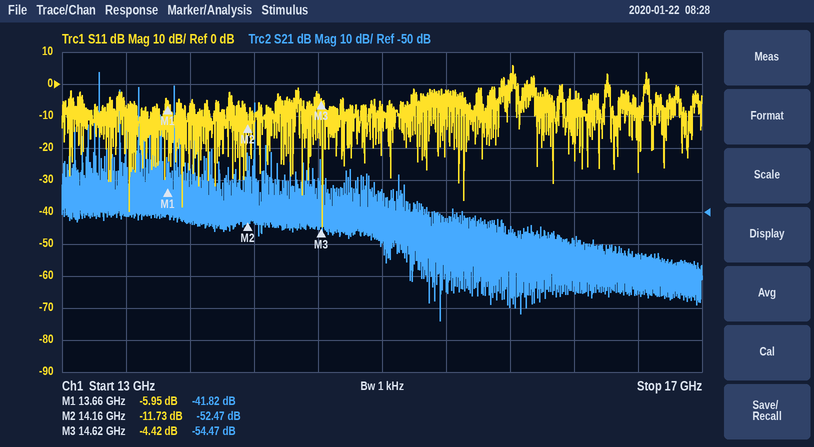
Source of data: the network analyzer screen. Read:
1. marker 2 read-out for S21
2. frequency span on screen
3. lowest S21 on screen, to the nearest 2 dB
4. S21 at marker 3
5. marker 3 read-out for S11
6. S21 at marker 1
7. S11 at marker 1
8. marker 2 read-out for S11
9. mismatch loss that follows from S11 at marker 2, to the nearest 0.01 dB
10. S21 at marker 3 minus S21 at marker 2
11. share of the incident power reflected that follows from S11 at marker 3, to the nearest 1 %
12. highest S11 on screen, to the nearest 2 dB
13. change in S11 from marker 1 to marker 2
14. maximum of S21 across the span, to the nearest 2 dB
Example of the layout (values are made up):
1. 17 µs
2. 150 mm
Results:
1. -52.47 dB
2. 4 GHz
3. -84 dB
4. -54.47 dB
5. -4.42 dB
6. -41.82 dB
7. -5.95 dB
8. -11.73 dB
9. 0.30 dB
10. -2.00 dB
11. 36 %
12. 6 dB
13. -5.78 dB
14. -6 dB
